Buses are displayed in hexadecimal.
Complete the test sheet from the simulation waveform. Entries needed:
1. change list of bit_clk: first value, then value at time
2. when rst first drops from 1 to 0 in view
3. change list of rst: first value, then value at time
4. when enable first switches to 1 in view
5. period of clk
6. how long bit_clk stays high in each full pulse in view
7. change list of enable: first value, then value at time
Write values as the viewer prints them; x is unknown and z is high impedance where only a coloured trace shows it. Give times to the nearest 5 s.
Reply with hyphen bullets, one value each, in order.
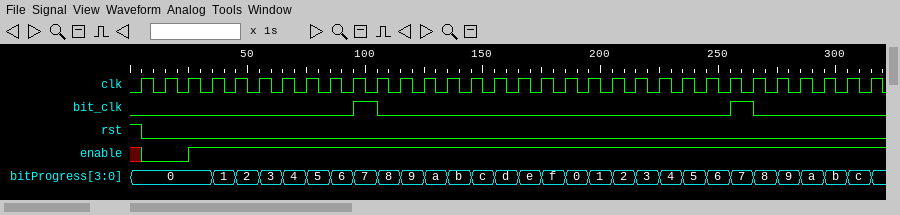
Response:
- 0, 1 at 95 s, 0 at 105 s, 1 at 255 s, 0 at 265 s
- 5 s
- 1, 0 at 5 s
- 25 s
- 10 s
- 10 s, 10 s
- x, 0 at 5 s, 1 at 25 s
